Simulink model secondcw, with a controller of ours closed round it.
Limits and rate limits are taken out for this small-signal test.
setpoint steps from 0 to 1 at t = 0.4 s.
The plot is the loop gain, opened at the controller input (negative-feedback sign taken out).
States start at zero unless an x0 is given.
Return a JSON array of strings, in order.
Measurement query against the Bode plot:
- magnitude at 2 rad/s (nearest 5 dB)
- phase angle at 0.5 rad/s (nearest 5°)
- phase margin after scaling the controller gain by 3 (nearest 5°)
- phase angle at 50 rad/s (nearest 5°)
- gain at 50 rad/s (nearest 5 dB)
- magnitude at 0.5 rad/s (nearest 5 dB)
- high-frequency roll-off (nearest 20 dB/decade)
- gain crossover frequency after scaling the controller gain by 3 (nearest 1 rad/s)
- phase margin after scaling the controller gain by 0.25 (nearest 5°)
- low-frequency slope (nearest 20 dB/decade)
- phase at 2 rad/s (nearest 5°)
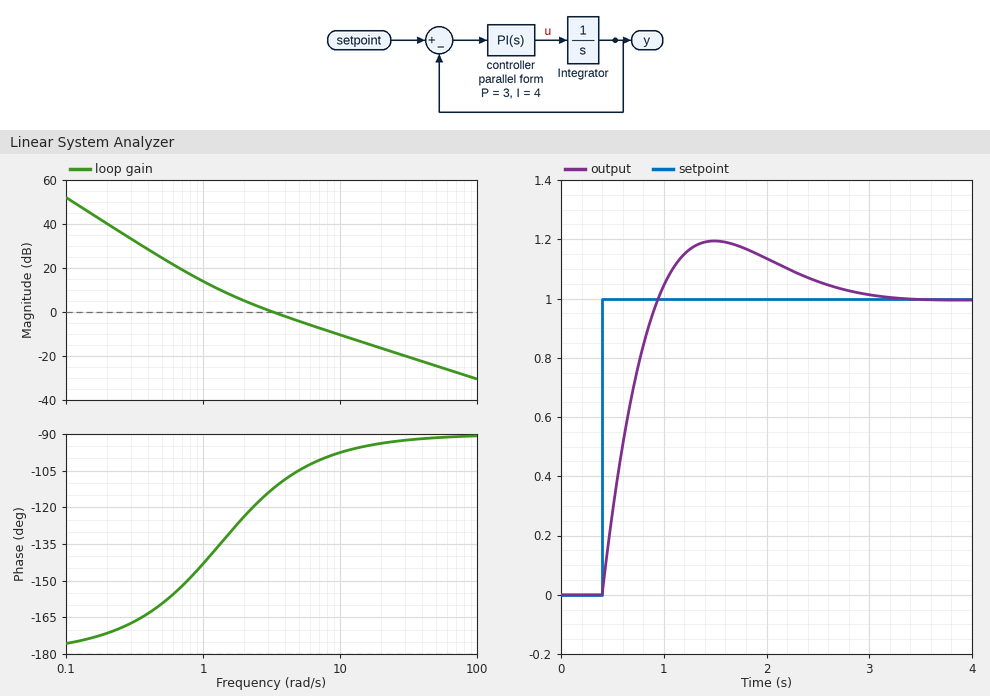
["5 dB", "-160°", "80°", "-90°", "-25 dB", "25 dB", "-20 dB/decade", "9 rad/s", "40°", "-40 dB/decade", "-125°"]
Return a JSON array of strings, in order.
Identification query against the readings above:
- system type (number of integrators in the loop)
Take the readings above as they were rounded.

["2"]
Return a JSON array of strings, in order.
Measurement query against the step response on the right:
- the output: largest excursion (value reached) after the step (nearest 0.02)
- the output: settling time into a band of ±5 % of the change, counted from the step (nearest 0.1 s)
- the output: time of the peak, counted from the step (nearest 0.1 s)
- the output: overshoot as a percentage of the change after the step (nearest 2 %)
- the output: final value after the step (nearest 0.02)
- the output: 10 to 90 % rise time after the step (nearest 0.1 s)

["1.20", "2.2 s", "1.1 s", "20 %", "1.00", "0.4 s"]
